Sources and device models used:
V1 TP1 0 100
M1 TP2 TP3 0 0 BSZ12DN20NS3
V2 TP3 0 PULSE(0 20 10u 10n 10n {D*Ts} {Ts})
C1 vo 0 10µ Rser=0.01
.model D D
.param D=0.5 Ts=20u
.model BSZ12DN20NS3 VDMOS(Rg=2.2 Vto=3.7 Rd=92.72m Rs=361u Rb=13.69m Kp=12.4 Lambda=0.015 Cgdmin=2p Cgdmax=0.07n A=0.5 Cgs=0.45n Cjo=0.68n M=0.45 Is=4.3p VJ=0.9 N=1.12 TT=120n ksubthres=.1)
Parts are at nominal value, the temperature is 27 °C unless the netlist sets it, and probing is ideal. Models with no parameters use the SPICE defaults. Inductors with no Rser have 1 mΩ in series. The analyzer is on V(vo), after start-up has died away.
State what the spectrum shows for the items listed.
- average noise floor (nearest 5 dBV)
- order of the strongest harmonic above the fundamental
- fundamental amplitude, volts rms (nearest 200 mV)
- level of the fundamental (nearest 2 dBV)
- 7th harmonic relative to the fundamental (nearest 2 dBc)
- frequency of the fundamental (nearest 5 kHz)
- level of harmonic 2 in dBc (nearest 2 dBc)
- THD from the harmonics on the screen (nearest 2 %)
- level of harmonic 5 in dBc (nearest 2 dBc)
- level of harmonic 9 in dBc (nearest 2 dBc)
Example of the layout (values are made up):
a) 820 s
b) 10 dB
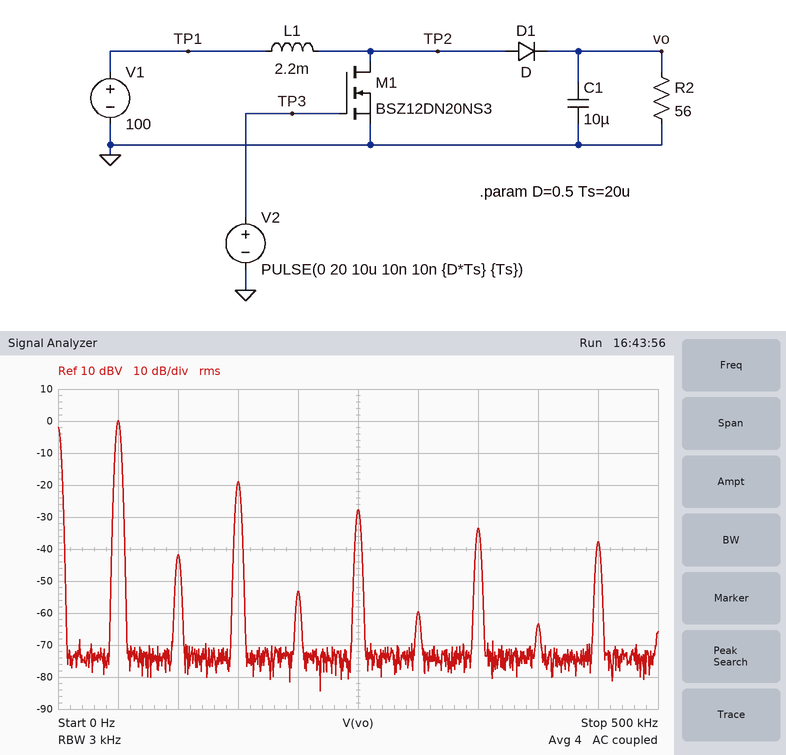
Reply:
a) -75 dBV
b) 3
c) 1.0 V
d) 0 dBV
e) -34 dBc
f) 50 kHz
g) -42 dBc
h) 12 %
i) -28 dBc
j) -38 dBc
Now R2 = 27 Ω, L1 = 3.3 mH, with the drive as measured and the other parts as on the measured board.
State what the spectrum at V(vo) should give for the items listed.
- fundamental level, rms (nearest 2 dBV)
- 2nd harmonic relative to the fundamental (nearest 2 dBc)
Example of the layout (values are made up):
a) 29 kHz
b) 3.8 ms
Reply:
a) 6 dBV
b) -50 dBc
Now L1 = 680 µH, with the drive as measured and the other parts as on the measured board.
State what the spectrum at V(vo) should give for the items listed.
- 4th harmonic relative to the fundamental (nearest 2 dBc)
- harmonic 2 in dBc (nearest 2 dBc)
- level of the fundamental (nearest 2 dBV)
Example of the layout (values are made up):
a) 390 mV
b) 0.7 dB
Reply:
a) -44 dBc
b) -32 dBc
c) 0 dBV
